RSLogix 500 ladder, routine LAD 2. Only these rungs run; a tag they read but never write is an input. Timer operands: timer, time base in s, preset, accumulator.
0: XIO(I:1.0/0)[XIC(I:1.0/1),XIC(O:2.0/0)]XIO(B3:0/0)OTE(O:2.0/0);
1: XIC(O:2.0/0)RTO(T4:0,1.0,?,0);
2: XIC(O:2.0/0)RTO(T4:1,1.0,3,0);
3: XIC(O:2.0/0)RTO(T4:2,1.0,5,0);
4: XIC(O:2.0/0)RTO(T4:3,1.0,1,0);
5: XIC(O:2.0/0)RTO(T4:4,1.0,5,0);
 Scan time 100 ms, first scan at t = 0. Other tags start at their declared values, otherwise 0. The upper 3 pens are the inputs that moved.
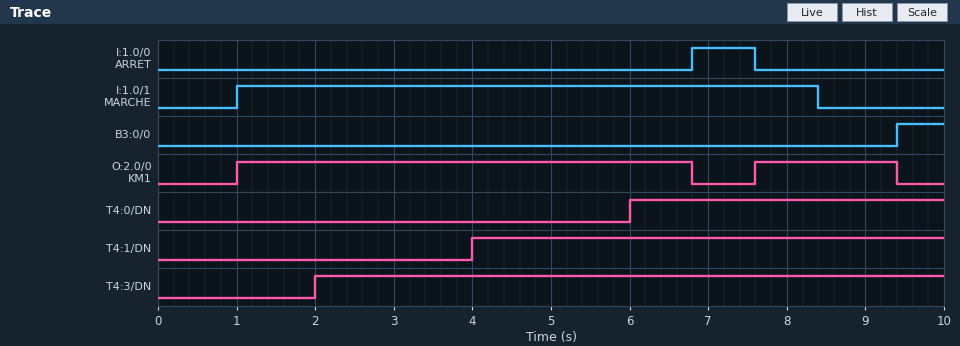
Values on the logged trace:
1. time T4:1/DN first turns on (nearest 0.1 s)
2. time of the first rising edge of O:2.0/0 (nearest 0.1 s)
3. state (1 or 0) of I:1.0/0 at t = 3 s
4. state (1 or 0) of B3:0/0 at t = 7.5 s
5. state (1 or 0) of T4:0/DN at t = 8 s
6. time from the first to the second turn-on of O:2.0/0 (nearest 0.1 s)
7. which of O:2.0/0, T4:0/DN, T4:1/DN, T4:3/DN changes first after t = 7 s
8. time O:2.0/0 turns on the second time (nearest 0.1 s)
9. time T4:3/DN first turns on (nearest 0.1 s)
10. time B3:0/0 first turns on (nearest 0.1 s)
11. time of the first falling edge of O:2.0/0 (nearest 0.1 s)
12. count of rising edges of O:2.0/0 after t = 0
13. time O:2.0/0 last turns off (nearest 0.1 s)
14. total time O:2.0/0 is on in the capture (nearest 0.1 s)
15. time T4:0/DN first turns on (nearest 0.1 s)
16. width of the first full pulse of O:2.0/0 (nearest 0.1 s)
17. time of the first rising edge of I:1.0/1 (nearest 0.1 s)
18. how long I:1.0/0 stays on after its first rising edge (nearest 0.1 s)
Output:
4.0 s
1.0 s
0
0
1
6.6 s
O:2.0/0
7.6 s
2.0 s
9.4 s
6.8 s
2
9.4 s
7.6 s
6.0 s
5.8 s
1.0 s
0.8 s
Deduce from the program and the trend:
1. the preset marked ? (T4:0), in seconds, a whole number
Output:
5 s
